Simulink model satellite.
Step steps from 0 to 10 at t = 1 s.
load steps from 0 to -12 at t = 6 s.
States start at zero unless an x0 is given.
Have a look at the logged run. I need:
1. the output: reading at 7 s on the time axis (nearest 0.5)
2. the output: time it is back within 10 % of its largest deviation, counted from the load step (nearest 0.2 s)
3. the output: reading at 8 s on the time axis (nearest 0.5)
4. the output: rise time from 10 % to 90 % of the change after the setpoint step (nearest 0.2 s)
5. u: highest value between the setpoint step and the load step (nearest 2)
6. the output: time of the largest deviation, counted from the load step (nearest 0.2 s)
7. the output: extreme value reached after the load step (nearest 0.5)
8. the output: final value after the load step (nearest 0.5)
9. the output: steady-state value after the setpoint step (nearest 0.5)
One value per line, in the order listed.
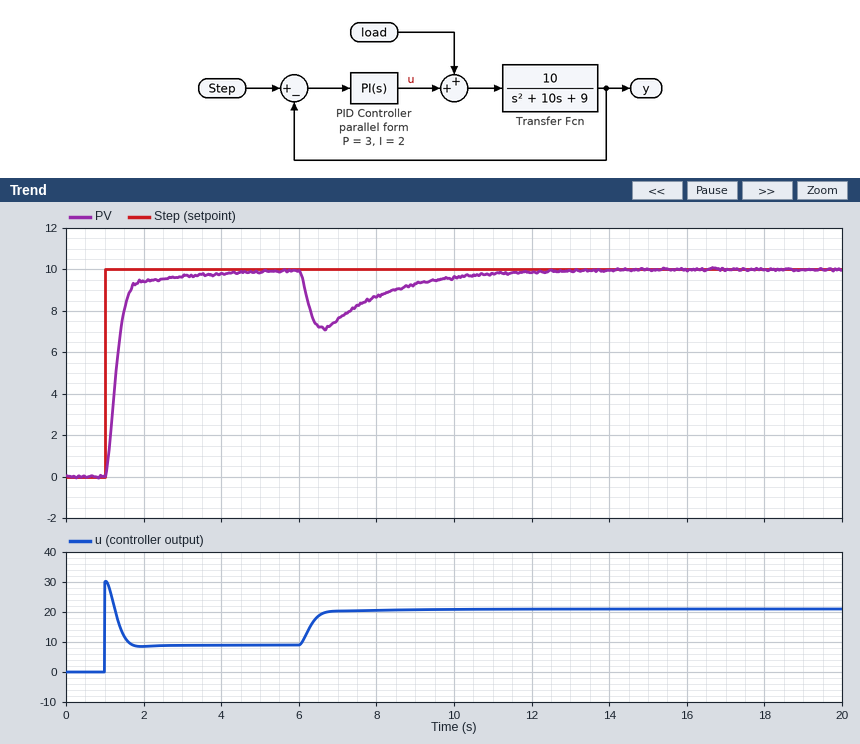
7.5
4.6 s
8.5
0.6 s
30
0.6 s
7.0
10.0
10.0
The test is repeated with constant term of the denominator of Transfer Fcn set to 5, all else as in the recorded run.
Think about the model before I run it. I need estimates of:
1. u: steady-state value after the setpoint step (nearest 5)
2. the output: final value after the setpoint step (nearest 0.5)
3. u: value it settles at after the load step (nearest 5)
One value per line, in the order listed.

5
10.0
15
